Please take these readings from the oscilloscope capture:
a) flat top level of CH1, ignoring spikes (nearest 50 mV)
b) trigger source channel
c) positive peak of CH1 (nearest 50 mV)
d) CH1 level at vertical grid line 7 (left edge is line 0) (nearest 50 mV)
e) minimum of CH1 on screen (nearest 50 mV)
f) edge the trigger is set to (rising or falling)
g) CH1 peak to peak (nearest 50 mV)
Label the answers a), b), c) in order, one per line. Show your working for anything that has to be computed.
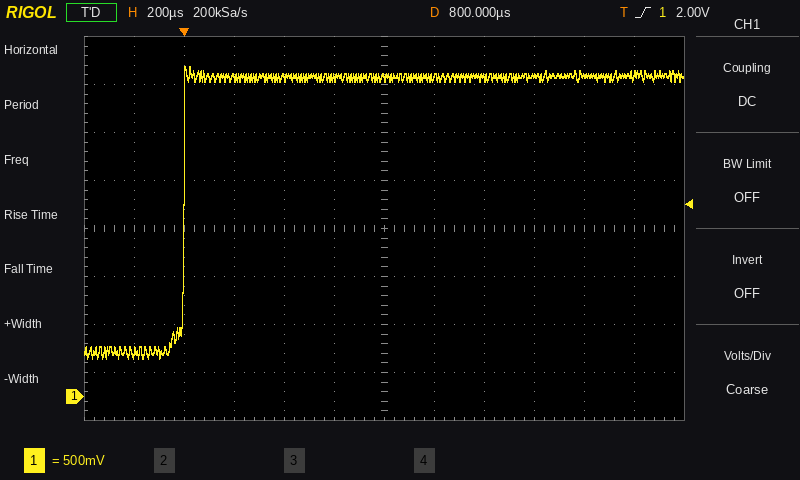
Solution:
a) 3.35 V
b) CH1
c) 3.45 V
d) 3.30 V
e) 400 mV
f) rising
g) 3.45 V − (400 mV) = 3.05 V
